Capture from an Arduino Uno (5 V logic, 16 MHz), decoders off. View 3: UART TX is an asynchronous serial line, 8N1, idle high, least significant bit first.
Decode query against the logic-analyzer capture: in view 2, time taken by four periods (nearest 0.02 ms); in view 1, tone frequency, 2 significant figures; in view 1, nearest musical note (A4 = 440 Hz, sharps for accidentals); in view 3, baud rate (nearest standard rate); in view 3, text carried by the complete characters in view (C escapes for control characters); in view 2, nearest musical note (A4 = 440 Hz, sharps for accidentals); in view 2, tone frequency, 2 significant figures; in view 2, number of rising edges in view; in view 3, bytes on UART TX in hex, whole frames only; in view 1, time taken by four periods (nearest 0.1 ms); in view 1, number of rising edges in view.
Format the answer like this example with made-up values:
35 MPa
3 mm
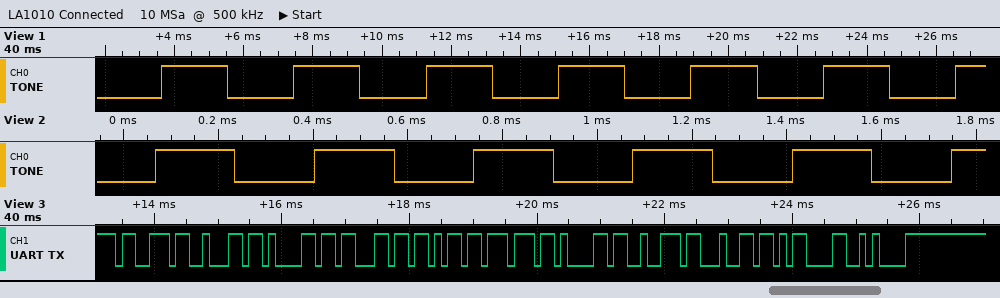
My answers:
1.34 ms
260 Hz
C4
9600 baud
"sbackward\r\n"
F#7
3.0 kHz
6
73 62 61 63 6B 77 61 72 64 0D 0A
15.3 ms
7
